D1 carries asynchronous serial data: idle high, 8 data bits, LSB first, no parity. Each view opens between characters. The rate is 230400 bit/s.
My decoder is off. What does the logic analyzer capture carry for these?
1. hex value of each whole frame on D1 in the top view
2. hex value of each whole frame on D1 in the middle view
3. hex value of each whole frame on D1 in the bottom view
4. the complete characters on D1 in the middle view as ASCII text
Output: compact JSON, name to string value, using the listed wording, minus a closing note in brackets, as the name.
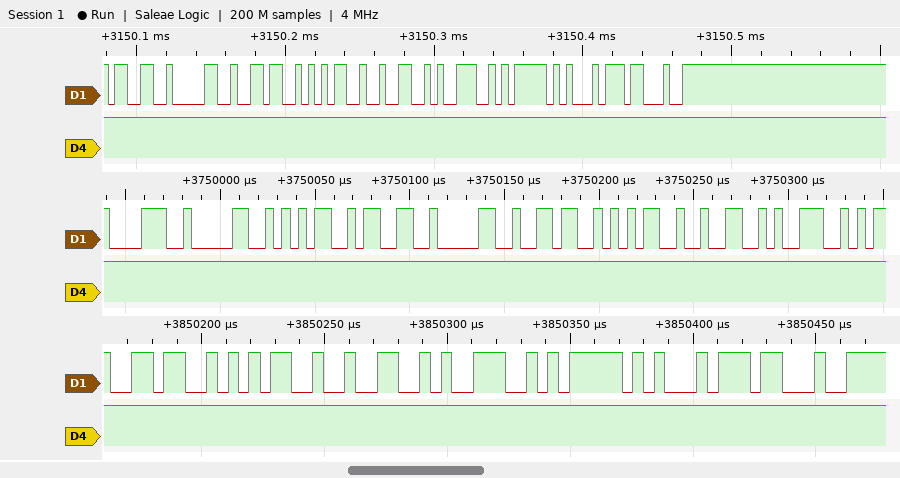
{"hex value of each whole frame on D1 in the top view": "33, 30, 36, 35, 32, 39, 7D, D1, 23", "hex value of each whole frame on D1 in the middle view": "38, 30, 35, 33, 30, 36, 35, 32, 39", "hex value of each whole frame on D1 in the bottom view": "36, 35, 32, 39, 7D, D1, 23", "the complete characters on D1 in the middle view as ASCII text": "\"805306529\""}
